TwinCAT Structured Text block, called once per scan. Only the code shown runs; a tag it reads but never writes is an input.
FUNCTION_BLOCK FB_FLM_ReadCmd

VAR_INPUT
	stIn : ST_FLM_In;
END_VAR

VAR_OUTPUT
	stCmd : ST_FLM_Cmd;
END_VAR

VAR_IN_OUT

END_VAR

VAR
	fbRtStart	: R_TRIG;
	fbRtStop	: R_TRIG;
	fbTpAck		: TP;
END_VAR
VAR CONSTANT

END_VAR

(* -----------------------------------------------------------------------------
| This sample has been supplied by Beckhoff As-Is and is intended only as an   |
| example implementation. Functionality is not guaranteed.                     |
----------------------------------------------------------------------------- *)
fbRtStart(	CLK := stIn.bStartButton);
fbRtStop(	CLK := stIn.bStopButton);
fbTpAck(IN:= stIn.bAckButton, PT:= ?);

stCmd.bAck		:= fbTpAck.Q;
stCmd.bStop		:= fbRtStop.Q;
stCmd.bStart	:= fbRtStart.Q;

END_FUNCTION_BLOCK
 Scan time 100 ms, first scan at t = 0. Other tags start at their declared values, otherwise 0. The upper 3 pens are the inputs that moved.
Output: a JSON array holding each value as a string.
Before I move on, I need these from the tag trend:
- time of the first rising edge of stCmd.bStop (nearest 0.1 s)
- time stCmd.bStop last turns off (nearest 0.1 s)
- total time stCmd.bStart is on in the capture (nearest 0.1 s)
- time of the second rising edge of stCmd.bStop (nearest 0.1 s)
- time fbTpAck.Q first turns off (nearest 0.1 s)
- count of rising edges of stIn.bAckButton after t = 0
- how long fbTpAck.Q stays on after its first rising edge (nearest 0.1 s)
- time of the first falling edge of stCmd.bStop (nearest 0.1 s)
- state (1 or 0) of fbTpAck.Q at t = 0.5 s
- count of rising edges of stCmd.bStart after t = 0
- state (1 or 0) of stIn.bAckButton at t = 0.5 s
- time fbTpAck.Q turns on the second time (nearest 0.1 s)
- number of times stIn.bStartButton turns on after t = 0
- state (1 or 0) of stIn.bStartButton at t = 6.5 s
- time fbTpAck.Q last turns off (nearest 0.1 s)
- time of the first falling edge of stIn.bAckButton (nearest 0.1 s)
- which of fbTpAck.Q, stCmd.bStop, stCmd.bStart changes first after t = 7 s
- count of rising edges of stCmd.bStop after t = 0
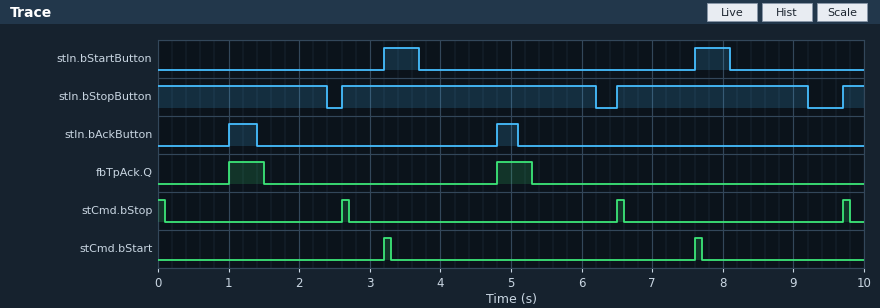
["2.6 s", "9.8 s", "0.2 s", "6.5 s", "1.5 s", "2", "0.5 s", "0.1 s", "0", "2", "0", "4.8 s", "2", "0", "5.3 s", "1.4 s", "stCmd.bStart", "3"]
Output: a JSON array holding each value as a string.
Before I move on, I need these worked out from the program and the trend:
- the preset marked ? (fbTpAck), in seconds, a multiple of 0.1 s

["0.5 s"]
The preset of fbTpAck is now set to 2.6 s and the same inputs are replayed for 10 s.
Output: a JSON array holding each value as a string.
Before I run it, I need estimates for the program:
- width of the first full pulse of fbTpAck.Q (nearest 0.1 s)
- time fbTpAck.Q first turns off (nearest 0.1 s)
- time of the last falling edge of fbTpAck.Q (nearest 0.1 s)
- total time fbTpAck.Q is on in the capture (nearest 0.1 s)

["2.6 s", "3.6 s", "7.4 s", "5.2 s"]
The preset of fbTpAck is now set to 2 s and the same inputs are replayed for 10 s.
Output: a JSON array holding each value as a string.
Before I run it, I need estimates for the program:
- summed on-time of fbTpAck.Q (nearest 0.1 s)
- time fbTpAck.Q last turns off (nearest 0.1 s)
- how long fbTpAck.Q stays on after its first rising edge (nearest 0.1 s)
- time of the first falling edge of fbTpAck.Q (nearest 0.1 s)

["4.0 s", "6.8 s", "2.0 s", "3.0 s"]
